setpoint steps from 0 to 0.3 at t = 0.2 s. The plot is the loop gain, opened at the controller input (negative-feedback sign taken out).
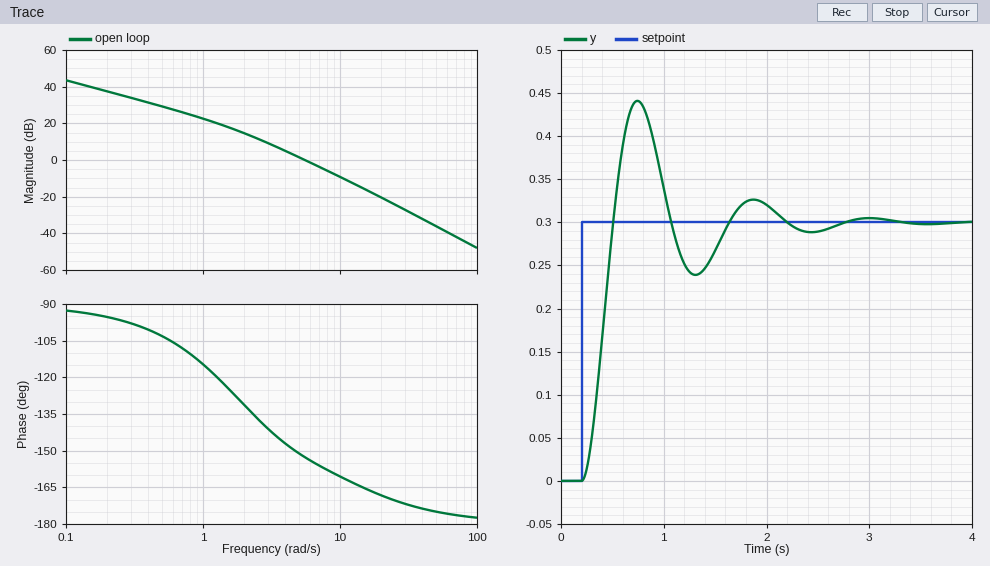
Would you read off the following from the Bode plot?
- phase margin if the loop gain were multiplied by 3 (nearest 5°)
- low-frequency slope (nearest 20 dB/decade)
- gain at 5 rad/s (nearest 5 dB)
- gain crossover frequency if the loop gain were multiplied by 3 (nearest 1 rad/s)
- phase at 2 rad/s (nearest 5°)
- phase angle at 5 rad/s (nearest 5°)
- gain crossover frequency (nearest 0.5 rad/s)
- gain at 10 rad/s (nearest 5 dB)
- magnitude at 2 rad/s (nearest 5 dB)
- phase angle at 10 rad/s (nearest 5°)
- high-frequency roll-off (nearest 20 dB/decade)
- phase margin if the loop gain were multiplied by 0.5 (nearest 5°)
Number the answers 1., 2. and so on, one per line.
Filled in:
1. 20°
2. -20 dB/decade
3. 0 dB
4. 10 rad/s
5. -130°
6. -150°
7. 5.5 rad/s
8. -10 dB
9. 15 dB
10. -160°
11. -40 dB/decade
12. 35°
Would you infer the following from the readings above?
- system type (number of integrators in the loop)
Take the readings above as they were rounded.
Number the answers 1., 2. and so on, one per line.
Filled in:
1. 1
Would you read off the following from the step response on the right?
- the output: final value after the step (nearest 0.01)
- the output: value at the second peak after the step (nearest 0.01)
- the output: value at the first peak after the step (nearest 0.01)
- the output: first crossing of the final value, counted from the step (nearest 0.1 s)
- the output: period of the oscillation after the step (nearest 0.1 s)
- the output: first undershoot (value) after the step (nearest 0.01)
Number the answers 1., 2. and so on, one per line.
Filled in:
1. 0.30
2. 0.33
3. 0.44
4. 0.3 s
5. 1.1 s
6. 0.24
